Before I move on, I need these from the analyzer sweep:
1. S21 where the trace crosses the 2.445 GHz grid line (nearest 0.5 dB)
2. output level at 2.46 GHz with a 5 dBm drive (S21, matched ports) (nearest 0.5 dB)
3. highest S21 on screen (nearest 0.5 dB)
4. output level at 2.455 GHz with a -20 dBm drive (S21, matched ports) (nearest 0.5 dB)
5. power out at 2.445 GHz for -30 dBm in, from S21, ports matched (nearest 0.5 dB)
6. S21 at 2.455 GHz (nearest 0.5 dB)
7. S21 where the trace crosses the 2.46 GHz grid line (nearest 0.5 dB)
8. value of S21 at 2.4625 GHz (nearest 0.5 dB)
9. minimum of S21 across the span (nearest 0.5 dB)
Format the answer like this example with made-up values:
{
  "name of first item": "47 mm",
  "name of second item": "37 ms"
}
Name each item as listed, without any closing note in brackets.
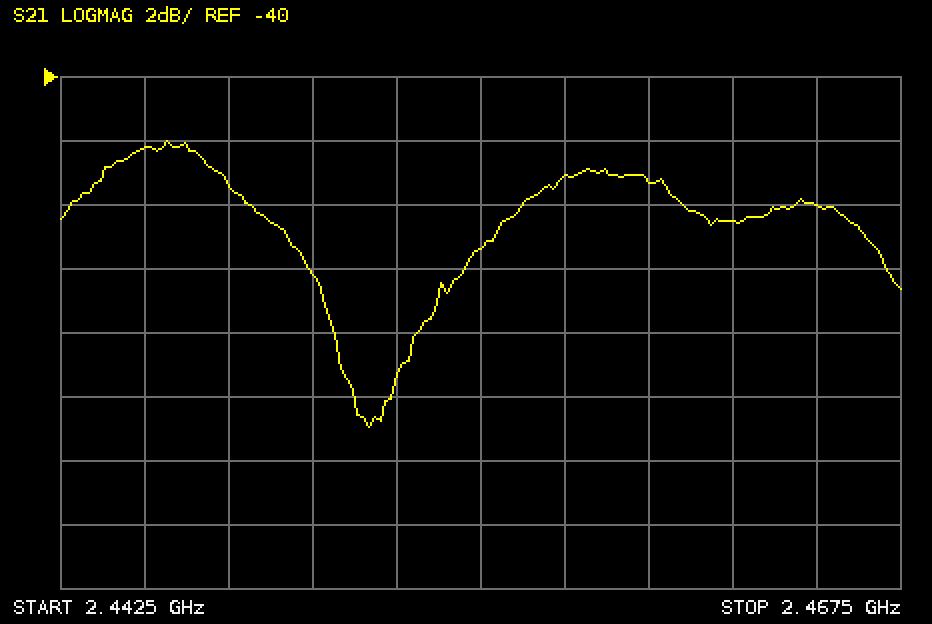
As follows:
{
  "S21 where the trace crosses the 2.445 GHz grid line": "-42.0 dB",
  "output level at 2.46 GHz with a 5 dBm drive (S21, matched ports)": "-38.5 dBm",
  "highest S21 on screen": "-42.0 dB",
  "output level at 2.455 GHz with a -20 dBm drive (S21, matched ports)": "-65.5 dBm",
  "power out at 2.445 GHz for -30 dBm in, from S21, ports matched": "-72.0 dBm",
  "S21 at 2.455 GHz": "-45.5 dB",
  "S21 where the trace crosses the 2.46 GHz grid line": "-43.5 dB",
  "value of S21 at 2.4625 GHz": "-44.5 dB",
  "minimum of S21 across the span": "-51.0 dB"
}
